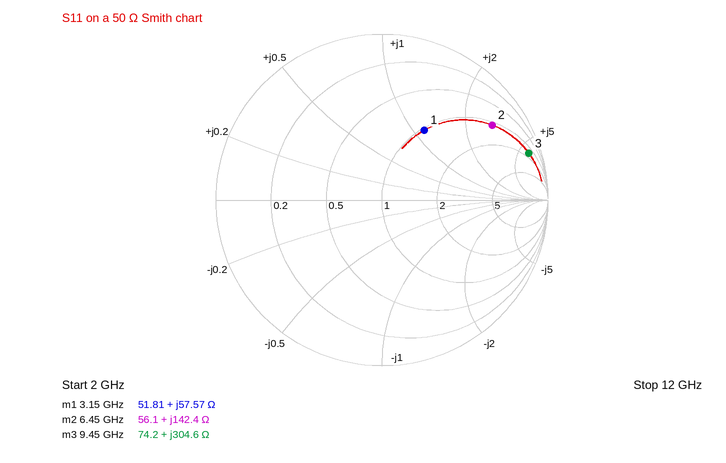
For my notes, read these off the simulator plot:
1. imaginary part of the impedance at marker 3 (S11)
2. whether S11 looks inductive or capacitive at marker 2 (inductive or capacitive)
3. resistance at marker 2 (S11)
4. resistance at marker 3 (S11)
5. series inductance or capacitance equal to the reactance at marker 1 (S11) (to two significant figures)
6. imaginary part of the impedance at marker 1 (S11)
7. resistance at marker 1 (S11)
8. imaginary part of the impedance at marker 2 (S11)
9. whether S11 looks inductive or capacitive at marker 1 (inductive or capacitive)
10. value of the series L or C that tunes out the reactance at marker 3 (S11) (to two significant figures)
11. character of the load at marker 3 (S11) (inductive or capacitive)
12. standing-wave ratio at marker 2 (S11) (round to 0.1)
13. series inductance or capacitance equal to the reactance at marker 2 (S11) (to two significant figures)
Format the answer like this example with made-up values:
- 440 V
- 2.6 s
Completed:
- +304.6 Ω
- inductive
- 56.1 Ω
- 74.2 Ω
- 2.9 nH
- +57.57 Ω
- 51.81 Ω
- +142.4 Ω
- inductive
- 55 fF
- inductive
- 9.1
- 3.5 nH
